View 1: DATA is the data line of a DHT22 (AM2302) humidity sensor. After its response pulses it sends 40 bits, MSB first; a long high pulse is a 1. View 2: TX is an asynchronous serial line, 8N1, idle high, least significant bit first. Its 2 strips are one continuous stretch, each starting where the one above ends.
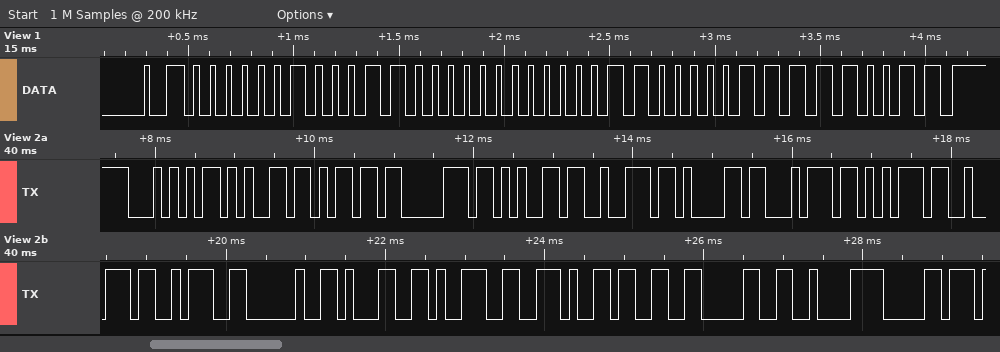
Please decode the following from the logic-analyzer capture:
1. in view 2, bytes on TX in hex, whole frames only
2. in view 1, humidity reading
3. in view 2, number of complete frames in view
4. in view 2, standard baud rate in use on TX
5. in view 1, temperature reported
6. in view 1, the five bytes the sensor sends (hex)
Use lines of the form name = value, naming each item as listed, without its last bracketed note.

in view 2, bytes on TX in hex, whole frames only = 54 65 6D 70 65 72 61 74 75 72 3A 20 31 39 2E 33 30 C2 B0
in view 1, humidity reading = 56.0 %
in view 2, number of complete frames in view = 19
in view 2, standard baud rate in use on TX = 9600 baud
in view 1, temperature reported = 19.3 °C
in view 1, the five bytes the sensor sends = 02 30 00 C1 F3
